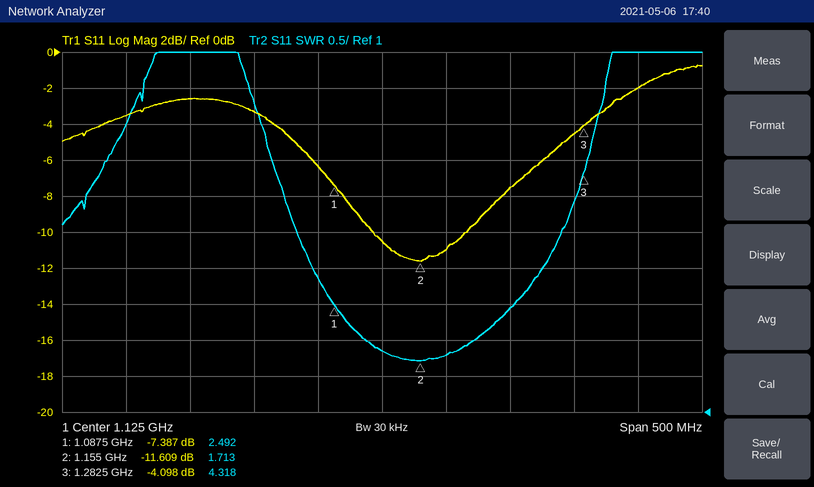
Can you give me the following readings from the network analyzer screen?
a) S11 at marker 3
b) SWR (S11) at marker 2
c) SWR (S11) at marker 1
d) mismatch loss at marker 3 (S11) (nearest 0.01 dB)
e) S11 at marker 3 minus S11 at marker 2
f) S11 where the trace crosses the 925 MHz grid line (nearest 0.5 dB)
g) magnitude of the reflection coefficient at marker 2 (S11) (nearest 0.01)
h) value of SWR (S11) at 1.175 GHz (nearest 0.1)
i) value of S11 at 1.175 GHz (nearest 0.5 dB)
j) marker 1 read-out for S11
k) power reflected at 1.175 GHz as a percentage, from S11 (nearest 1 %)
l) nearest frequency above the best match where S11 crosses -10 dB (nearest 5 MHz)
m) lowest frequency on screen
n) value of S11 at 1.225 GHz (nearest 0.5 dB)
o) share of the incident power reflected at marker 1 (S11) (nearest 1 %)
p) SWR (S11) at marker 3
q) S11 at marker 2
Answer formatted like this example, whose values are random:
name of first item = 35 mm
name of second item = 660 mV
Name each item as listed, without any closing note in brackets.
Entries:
S11 at marker 3 = -4.098 dB
SWR (S11) at marker 2 = 1.713
SWR (S11) at marker 1 = 2.492
mismatch loss at marker 3 (S11) = 2.14 dB
S11 at marker 3 minus S11 at marker 2 = 7.511 dB
S11 where the trace crosses the 925 MHz grid line = -3.5 dB
magnitude of the reflection coefficient at marker 2 (S11) = 0.26
value of SWR (S11) at 1.175 GHz = 1.8
value of S11 at 1.175 GHz = -11.0 dB
marker 1 read-out for S11 = -7.387 dB
power reflected at 1.175 GHz as a percentage, from S11 = 8 %
nearest frequency above the best match where S11 crosses -10 dB = 1.190 GHz
lowest frequency on screen = 875 MHz
value of S11 at 1.225 GHz = -7.5 dB
share of the incident power reflected at marker 1 (S11) = 18 %
SWR (S11) at marker 3 = 4.318
S11 at marker 2 = -11.609 dB
